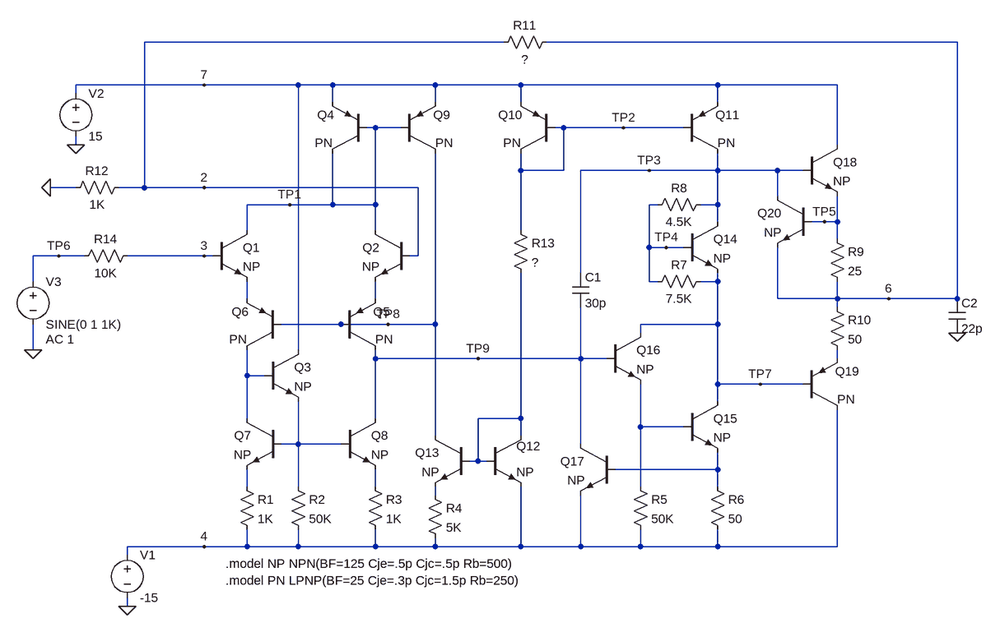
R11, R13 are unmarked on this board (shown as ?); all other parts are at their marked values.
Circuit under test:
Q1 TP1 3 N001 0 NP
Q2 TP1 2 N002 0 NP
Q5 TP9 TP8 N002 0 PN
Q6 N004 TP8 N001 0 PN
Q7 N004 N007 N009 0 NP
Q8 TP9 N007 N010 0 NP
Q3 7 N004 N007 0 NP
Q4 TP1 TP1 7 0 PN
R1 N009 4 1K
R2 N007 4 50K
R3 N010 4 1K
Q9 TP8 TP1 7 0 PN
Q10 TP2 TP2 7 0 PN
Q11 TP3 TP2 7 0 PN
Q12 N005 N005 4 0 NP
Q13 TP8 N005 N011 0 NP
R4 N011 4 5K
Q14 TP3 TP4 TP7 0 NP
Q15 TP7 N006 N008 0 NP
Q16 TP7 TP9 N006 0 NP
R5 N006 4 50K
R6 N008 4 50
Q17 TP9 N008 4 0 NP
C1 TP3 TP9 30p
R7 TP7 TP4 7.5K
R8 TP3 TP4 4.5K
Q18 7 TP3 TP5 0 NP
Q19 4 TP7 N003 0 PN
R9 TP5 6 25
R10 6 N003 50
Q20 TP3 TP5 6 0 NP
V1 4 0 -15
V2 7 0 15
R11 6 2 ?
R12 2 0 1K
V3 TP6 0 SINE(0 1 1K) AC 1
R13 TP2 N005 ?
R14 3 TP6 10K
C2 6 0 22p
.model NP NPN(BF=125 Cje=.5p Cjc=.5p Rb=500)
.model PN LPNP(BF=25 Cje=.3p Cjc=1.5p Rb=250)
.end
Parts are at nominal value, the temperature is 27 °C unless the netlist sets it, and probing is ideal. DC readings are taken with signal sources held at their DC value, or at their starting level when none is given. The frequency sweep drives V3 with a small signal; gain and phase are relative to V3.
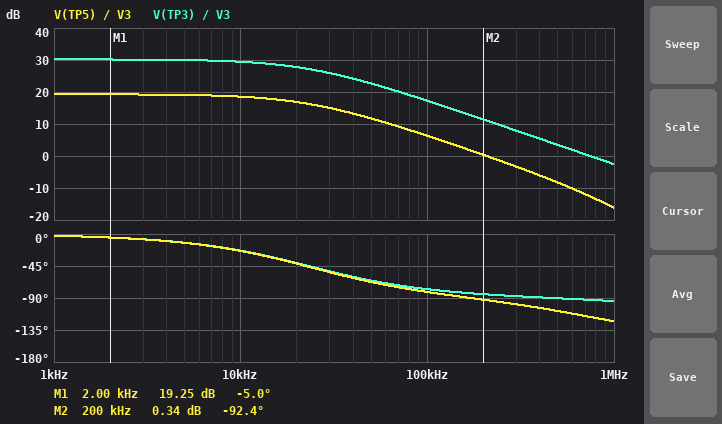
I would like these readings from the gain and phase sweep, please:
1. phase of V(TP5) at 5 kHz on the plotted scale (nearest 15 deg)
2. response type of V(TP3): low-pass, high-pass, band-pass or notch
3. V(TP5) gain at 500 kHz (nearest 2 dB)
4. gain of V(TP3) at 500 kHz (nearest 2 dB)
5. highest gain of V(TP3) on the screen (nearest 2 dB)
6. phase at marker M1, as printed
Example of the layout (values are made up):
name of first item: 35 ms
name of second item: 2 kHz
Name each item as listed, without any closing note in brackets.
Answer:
phase of V(TP5) at 5 kHz on the plotted scale: -15 deg
response type of V(TP3): low-pass, high-pass, band-pass or notch: low-pass
V(TP5) gain at 500 kHz: -8 dB
gain of V(TP3) at 500 kHz: 4 dB
highest gain of V(TP3) on the screen: 30 dB
phase at marker M1, as printed: -5.0 deg
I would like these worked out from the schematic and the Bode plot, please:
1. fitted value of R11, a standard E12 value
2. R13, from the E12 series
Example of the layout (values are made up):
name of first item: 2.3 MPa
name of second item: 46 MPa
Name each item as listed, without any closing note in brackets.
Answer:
fitted value of R11, a standard E12 value: 8.2 kΩ
R13, from the E12 series: 120 kΩ
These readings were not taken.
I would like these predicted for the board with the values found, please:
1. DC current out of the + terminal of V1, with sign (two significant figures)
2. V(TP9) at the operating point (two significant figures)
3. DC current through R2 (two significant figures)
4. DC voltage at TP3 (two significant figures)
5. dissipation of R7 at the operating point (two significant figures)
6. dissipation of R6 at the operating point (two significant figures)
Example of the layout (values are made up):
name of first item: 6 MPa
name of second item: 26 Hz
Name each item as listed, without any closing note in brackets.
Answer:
DC current out of the + terminal of V1, with sign: -500 µA
V(TP9) at the operating point: -14 V
DC current through R2: 13 µA
DC voltage at TP3: 570 mV
dissipation of R7 at the operating point: 69 µW
dissipation of R6 at the operating point: 2.1 µW
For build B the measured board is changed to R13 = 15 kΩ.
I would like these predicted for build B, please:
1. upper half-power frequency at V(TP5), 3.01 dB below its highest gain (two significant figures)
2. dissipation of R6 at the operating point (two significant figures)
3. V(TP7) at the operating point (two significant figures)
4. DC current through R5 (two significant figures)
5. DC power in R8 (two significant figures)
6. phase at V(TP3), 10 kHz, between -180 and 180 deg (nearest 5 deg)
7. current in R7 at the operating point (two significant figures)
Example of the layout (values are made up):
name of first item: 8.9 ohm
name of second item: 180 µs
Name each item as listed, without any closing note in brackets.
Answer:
upper half-power frequency at V(TP5), 3.01 dB below its highest gain: 120 kHz
dissipation of R6 at the operating point: 150 µW
V(TP7) at the operating point: -670 mV
DC current through R5: 18 µA
DC power in R8: 64 µW
phase at V(TP3), 10 kHz, between -180 and 180 deg: -5 deg
current in R7 at the operating point: 110 µA
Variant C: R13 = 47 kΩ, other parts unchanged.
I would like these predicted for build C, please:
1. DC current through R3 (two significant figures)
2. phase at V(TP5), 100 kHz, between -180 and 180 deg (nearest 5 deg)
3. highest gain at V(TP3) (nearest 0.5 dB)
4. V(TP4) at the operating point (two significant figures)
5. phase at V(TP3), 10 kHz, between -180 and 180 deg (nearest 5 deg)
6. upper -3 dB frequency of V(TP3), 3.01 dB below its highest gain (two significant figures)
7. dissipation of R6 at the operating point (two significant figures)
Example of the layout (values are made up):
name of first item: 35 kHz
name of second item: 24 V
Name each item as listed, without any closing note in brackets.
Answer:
DC current through R3: 9.2 µA
phase at V(TP5), 100 kHz, between -180 and 180 deg: -60 deg
highest gain at V(TP3): 24.0 dB
V(TP4) at the operating point: 140 mV
phase at V(TP3), 10 kHz, between -180 and 180 deg: -10 deg
upper -3 dB frequency of V(TP3), 3.01 dB below its highest gain: 61 kHz
dissipation of R6 at the operating point: 15 µW
